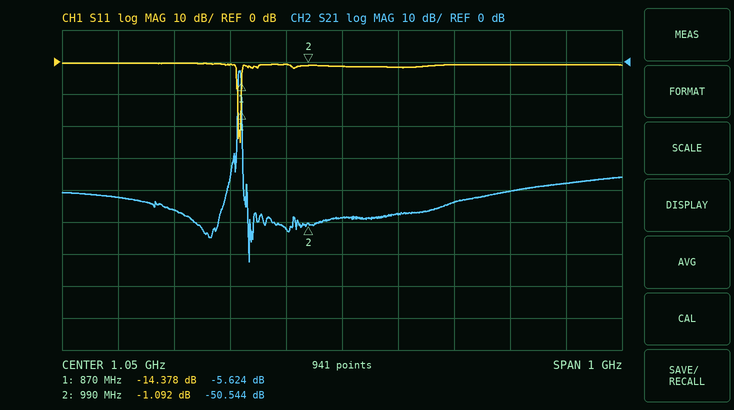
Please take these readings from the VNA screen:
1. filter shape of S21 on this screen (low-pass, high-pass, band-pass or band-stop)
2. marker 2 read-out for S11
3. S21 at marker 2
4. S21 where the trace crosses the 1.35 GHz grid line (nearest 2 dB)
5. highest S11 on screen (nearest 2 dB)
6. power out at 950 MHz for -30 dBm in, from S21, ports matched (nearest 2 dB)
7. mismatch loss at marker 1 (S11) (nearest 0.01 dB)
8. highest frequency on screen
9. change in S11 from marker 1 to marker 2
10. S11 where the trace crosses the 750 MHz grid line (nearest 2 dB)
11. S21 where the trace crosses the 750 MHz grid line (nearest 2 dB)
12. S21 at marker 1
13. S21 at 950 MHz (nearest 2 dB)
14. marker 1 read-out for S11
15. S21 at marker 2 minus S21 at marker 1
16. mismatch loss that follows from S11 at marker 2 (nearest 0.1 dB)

band-pass
-1.092 dB
-50.544 dB
-40 dB
0 dB
-82 dBm
0.16 dB
1.55 GHz
13.286 dB
0 dB
-46 dB
-5.624 dB
-52 dB
-14.378 dB
-44.920 dB
6.5 dB
